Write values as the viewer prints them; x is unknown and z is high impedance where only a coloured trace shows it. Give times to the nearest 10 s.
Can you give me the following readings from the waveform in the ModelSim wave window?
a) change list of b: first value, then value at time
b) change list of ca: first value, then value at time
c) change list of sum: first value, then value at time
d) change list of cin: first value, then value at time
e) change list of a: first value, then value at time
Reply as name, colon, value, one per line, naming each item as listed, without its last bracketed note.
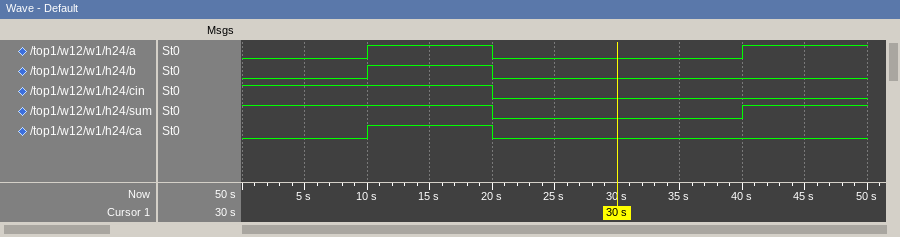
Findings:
change list of b: first value, then value at time: 0, 1 at 10 s, 0 at 20 s
change list of ca: first value, then value at time: 0, 1 at 10 s, 0 at 20 s
change list of sum: first value, then value at time: 1, 0 at 20 s, 1 at 40 s
change list of cin: first value, then value at time: 1, 0 at 20 s
change list of a: first value, then value at time: 0, 1 at 10 s, 0 at 20 s, 1 at 40 s
